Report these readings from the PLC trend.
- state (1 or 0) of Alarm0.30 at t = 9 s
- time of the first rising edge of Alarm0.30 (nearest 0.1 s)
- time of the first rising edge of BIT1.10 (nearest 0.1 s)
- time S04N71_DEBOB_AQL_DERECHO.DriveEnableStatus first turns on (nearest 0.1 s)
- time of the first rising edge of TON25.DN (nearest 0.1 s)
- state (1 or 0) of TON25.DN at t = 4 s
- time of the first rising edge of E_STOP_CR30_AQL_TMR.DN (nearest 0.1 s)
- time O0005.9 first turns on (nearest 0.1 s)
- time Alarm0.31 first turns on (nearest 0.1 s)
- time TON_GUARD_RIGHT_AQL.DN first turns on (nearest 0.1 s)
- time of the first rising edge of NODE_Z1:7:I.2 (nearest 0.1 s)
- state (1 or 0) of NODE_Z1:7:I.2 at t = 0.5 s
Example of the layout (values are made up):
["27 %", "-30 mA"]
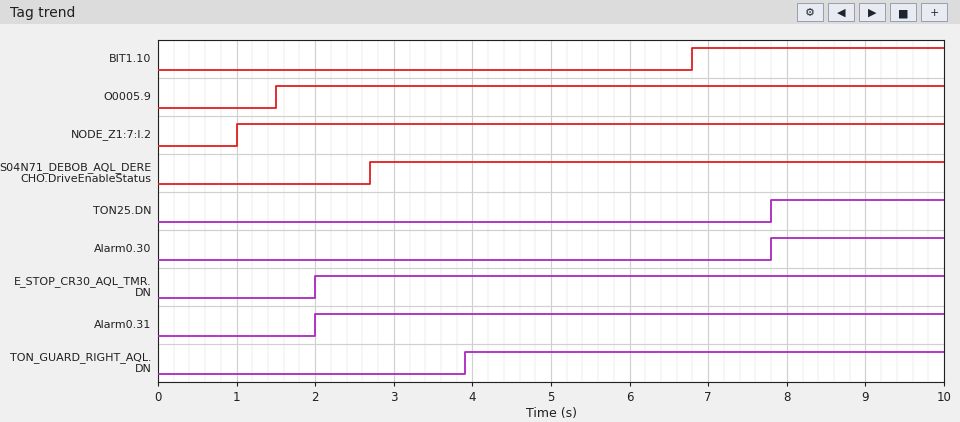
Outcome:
["1", "7.8 s", "6.8 s", "2.7 s", "7.8 s", "0", "2.0 s", "1.5 s", "2.0 s", "3.9 s", "1.0 s", "0"]
